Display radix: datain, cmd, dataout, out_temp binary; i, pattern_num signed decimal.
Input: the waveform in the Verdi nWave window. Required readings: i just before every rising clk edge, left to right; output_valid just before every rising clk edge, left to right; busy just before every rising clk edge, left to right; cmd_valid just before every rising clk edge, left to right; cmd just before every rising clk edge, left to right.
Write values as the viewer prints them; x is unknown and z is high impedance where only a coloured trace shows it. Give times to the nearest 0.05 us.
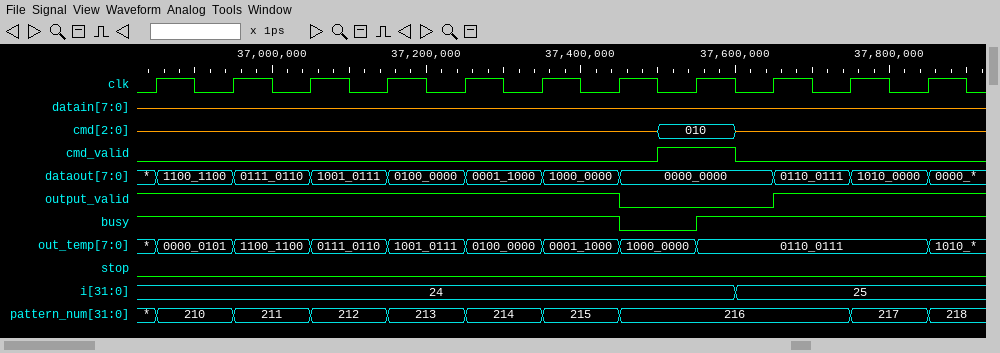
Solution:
24, 24, 24, 24, 24, 24, 24, 24, 25, 25, 25
1 1 1 1 1 1 1 0 0 1 1
1 1 1 1 1 1 1 0 1 1 1
0 0 0 0 0 0 0 1 0 0 0
z, z, z, z, z, z, z, 010, z, z, z
